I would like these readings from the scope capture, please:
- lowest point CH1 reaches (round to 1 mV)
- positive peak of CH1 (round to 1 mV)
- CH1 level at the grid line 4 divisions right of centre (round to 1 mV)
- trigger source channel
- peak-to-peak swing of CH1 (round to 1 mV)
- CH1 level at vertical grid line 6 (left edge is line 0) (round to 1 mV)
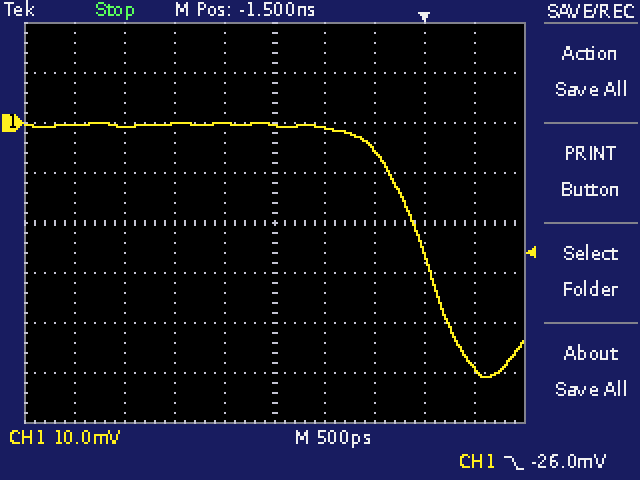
-51 mV
0 mV
-49 mV
CH1
51 mV
-1 mV
